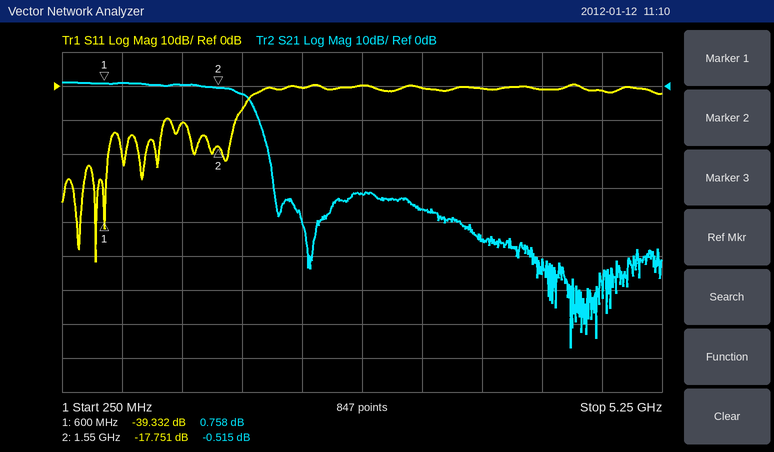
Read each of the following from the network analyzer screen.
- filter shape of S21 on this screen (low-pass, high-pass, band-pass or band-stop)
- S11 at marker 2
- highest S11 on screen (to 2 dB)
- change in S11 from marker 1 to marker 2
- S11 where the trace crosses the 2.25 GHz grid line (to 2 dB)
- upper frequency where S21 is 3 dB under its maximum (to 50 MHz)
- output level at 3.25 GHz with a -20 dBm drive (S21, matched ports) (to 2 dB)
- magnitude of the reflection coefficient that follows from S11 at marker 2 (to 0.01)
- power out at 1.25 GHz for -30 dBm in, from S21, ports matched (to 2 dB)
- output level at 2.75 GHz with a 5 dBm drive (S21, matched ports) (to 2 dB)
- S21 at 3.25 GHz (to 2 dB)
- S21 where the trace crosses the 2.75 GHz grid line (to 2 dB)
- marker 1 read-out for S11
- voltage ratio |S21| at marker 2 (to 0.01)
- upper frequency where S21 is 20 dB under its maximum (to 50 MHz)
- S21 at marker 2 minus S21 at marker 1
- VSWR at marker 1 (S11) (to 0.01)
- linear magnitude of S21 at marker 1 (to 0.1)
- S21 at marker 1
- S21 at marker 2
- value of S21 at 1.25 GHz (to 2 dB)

low-pass
-17.751 dB
0 dB
21.581 dB
0 dB
1.70 GHz
-56 dBm
0.13
-30 dBm
-26 dBm
-36 dB
-32 dB
-39.332 dB
0.94
1.95 GHz
-1.273 dB
1.02
1.1
0.758 dB
-0.515 dB
0 dB
